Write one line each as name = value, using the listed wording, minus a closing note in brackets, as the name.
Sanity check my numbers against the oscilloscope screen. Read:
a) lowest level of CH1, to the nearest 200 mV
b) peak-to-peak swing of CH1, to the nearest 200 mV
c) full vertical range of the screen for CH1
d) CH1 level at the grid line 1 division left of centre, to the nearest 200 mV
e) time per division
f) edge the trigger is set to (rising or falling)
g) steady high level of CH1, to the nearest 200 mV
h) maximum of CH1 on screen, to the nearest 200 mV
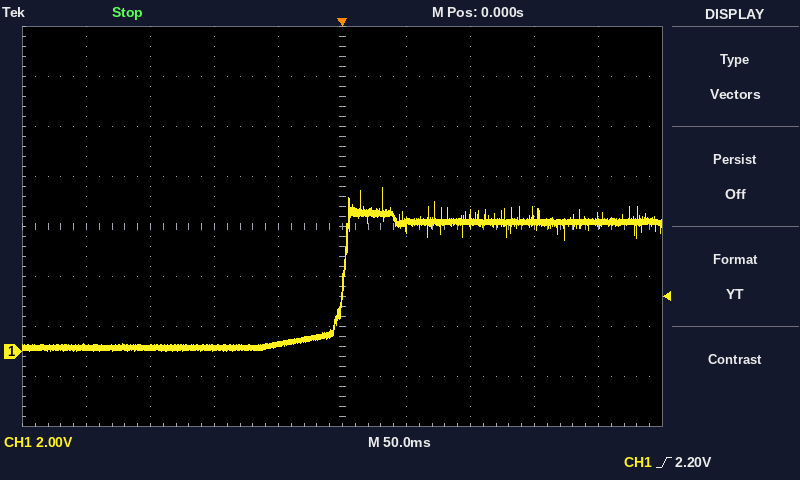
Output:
lowest level of CH1, to the nearest 200 mV = 0.0 V
peak-to-peak swing of CH1, to the nearest 200 mV = 6.6 V
full vertical range of the screen for CH1 = 16 V
CH1 level at the grid line 1 division left of centre, to the nearest 200 mV = 200 mV
time per division = 50 ms
edge the trigger is set to = rising
steady high level of CH1, to the nearest 200 mV = 5.2 V
maximum of CH1 on screen, to the nearest 200 mV = 6.6 V
